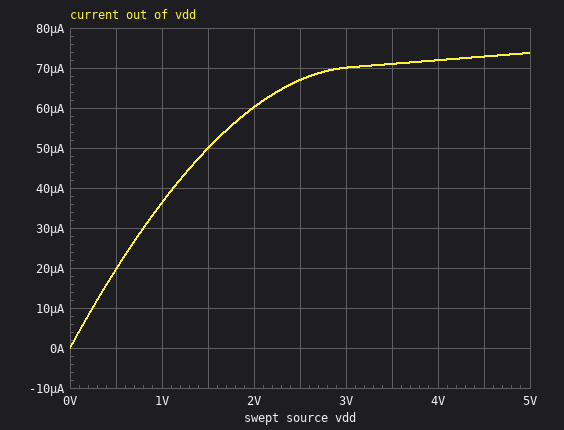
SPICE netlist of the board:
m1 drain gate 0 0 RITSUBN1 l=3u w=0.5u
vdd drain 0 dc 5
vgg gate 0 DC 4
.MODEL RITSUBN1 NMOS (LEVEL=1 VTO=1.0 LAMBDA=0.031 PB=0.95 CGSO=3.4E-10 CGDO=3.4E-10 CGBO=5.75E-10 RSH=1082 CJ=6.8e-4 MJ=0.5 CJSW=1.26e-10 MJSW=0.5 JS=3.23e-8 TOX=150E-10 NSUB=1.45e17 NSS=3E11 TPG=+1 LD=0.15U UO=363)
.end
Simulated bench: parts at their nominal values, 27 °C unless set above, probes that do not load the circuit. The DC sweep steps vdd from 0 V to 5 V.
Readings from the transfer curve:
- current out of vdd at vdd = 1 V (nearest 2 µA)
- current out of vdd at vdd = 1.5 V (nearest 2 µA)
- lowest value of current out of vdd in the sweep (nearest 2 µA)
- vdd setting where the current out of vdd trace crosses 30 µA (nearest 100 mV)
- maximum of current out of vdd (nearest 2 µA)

36 µA
50 µA
0 A
800 mV
74 µA
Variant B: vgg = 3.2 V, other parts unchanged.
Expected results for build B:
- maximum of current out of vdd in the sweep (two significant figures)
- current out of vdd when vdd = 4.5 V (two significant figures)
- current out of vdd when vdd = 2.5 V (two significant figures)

41 µA
40 µA
38 µA
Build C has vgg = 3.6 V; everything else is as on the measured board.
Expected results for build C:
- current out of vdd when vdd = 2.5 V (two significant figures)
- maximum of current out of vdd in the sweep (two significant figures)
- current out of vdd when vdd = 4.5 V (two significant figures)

52 µA
56 µA
55 µA
